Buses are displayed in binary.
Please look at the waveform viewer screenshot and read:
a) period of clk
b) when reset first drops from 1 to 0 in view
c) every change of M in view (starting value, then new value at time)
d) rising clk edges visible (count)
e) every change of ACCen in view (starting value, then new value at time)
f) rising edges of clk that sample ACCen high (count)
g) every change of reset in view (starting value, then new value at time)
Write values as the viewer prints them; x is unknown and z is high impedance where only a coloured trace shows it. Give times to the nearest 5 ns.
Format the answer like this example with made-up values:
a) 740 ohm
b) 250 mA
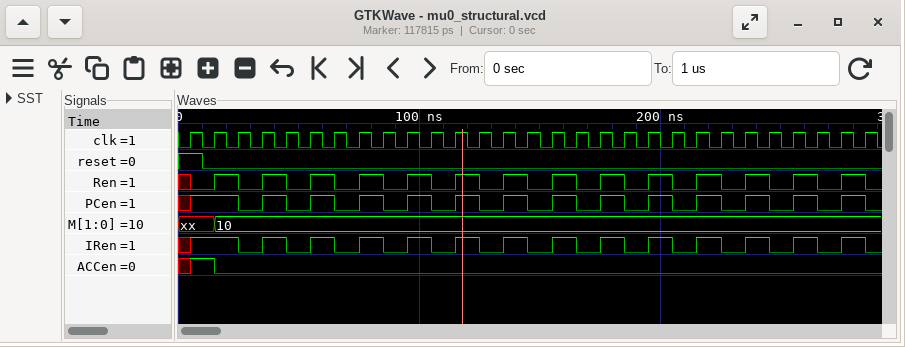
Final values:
a) 10 ns
b) 10 ns
c) xx, 10 at 15 ns
d) 29
e) x, 1 at 5 ns, 0 at 15 ns
f) 1
g) 1, 0 at 10 ns
